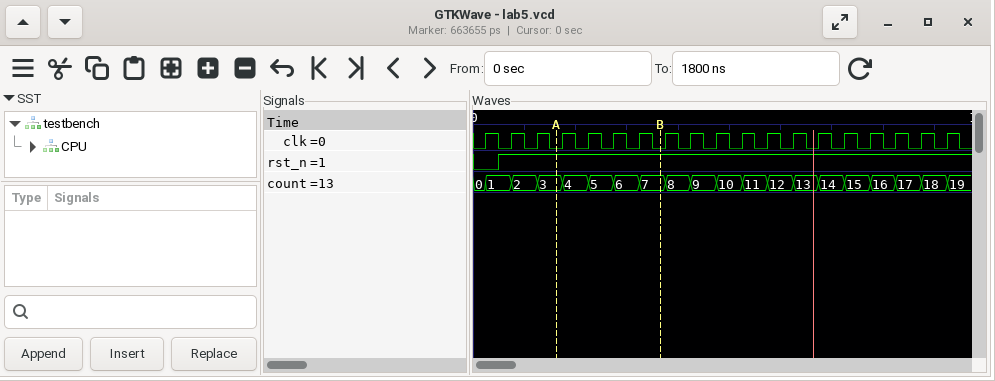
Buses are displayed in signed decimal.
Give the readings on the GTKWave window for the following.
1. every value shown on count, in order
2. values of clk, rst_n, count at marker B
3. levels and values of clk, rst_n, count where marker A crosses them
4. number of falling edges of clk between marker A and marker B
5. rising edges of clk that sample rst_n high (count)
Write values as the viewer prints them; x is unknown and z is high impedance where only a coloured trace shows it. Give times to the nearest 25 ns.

0, 1, 2, 3, 4, 5, 6, 7, 8, 9, 10, 11, 12, 13, 14, 15, 16, 17, 18, 19
clk=0, rst_n=1, count=7
clk=0, rst_n=1, count=3
4
18
